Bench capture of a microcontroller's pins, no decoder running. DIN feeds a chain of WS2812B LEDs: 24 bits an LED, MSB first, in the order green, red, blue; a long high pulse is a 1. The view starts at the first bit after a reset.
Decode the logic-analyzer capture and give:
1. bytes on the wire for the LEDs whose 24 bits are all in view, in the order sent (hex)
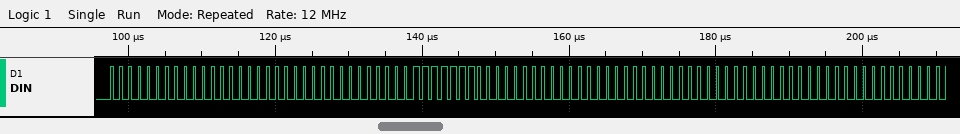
00 00 00 00 7F 00 00 00 00
